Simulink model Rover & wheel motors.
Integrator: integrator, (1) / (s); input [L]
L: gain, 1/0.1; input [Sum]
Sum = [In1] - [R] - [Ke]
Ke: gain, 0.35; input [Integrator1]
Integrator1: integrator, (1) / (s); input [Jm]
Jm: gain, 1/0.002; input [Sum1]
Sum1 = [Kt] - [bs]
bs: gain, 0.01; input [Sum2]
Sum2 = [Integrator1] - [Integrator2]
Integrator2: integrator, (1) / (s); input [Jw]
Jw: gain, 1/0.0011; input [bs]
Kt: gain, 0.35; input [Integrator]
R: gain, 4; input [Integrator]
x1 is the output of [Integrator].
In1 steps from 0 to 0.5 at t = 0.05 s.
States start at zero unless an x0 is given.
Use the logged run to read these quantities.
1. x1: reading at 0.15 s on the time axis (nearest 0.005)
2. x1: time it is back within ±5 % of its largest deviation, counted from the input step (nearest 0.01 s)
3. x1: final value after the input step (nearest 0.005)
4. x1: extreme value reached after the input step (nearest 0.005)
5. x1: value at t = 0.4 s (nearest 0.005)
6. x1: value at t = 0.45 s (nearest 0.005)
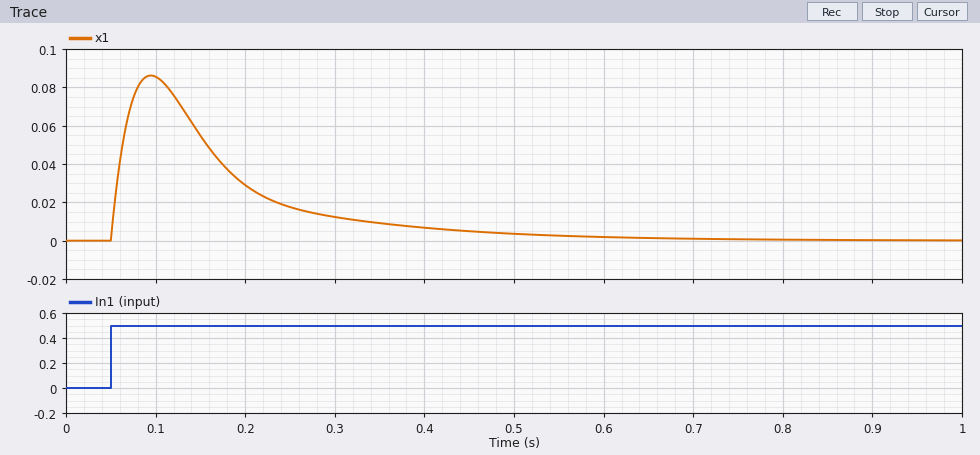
0.055
0.42 s
0.000
0.085
0.005
0.005
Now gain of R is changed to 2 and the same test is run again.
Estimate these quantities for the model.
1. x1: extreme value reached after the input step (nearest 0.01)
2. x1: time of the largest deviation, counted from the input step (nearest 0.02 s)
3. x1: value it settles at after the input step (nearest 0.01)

0.12
0.06 s
0.00
